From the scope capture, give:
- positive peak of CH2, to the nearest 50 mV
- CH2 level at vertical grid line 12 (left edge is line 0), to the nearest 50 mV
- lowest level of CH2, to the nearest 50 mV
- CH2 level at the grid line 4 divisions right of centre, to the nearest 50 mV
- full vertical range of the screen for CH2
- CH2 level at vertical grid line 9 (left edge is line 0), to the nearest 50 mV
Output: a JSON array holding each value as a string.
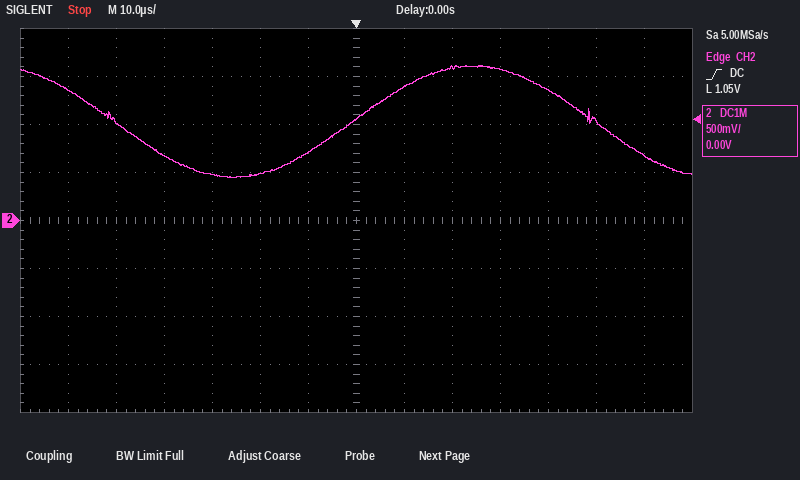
["1.60 V", "1.05 V", "450 mV", "1.35 V", "4 V", "1.60 V"]
